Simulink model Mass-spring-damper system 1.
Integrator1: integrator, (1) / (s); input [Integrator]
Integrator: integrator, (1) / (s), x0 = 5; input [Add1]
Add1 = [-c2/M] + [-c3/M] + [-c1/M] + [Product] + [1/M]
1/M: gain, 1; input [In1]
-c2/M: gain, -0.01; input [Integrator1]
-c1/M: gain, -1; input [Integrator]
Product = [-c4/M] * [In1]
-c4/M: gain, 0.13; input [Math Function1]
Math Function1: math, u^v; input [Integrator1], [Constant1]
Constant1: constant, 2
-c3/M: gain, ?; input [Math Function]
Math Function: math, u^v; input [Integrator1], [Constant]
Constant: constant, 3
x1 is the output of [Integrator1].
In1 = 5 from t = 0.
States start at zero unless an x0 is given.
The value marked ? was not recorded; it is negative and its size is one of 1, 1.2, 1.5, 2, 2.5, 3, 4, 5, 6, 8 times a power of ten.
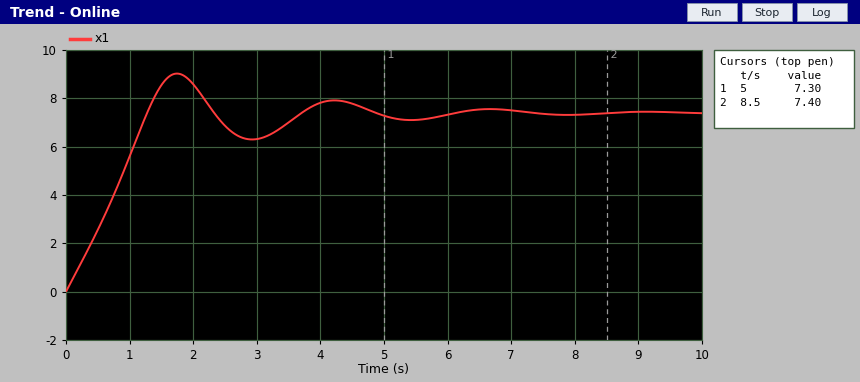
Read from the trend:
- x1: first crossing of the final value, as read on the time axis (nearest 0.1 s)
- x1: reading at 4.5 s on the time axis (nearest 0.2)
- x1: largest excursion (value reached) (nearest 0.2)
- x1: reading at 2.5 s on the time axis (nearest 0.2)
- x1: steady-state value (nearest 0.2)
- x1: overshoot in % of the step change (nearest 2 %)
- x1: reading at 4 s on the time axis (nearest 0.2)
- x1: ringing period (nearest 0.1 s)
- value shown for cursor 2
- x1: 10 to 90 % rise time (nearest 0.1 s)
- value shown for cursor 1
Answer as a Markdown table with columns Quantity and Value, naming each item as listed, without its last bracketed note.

| Quantity | Value |
|---|---|
| x1: first crossing of the final value, as read on the time axis | 1.3 s |
| x1: reading at 4.5 s on the time axis | 7.8 |
| x1: largest excursion (value reached) | 9.0 |
| x1: reading at 2.5 s on the time axis | 6.8 |
| x1: steady-state value | 7.4 |
| x1: overshoot in % of the step change | 22 % |
| x1: reading at 4 s on the time axis | 7.8 |
| x1: ringing period | 2.5 s |
| value shown for cursor 2 | 7.40 |
| x1: 10 to 90 % rise time | 1.0 s |
| value shown for cursor 1 | 7.30 |
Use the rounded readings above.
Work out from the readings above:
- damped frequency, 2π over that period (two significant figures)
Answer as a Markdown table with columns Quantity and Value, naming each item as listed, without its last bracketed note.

| Quantity | Value |
|---|---|
| damped frequency, 2π over that period | 2.5 rad/s |
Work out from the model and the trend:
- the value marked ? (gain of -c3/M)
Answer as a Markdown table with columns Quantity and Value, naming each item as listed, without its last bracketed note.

| Quantity | Value |
|---|---|
| the value marked ? | -0.1 |
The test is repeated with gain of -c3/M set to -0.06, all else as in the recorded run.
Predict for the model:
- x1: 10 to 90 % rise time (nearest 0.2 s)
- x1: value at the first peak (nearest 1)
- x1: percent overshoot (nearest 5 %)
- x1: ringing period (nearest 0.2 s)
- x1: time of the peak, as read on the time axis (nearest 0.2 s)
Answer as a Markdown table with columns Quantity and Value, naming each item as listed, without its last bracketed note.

| Quantity | Value |
|---|---|
| x1: 10 to 90 % rise time | 1.2 s |
| x1: value at the first peak | 14 |
| x1: percent overshoot | 20 % |
| x1: ringing period | 2.2 s |
| x1: time of the peak, as read on the time axis | 2.0 s |
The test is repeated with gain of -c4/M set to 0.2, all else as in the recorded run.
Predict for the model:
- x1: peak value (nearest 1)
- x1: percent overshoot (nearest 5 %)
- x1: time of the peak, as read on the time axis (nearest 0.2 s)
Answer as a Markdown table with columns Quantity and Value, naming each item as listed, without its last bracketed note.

| Quantity | Value |
|---|---|
| x1: peak value | 13 |
| x1: percent overshoot | 20 % |
| x1: time of the peak, as read on the time axis | 1.8 s |
